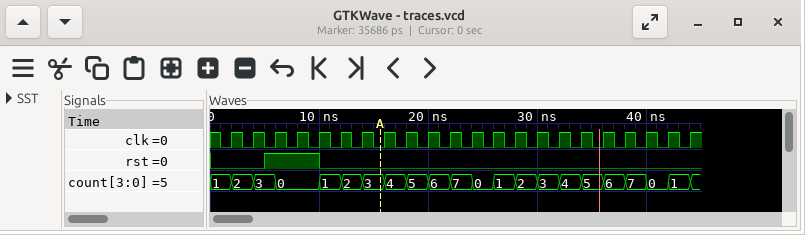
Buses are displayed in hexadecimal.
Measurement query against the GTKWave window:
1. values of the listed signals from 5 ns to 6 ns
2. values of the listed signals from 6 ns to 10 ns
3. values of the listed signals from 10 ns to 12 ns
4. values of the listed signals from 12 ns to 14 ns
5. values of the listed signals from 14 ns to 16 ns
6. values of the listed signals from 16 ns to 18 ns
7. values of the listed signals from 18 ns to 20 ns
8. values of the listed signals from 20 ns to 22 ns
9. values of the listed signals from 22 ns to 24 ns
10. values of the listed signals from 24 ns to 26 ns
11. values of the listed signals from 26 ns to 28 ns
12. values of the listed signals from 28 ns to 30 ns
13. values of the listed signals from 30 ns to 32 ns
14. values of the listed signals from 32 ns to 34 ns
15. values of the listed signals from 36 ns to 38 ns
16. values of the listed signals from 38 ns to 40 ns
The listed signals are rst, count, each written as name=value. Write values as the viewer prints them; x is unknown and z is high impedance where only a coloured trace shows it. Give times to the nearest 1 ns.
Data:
rst=1, count=3
rst=1, count=0
rst=0, count=1
rst=0, count=2
rst=0, count=3
rst=0, count=4
rst=0, count=5
rst=0, count=6
rst=0, count=7
rst=0, count=0
rst=0, count=1
rst=0, count=2
rst=0, count=3
rst=0, count=4
rst=0, count=6
rst=0, count=7
